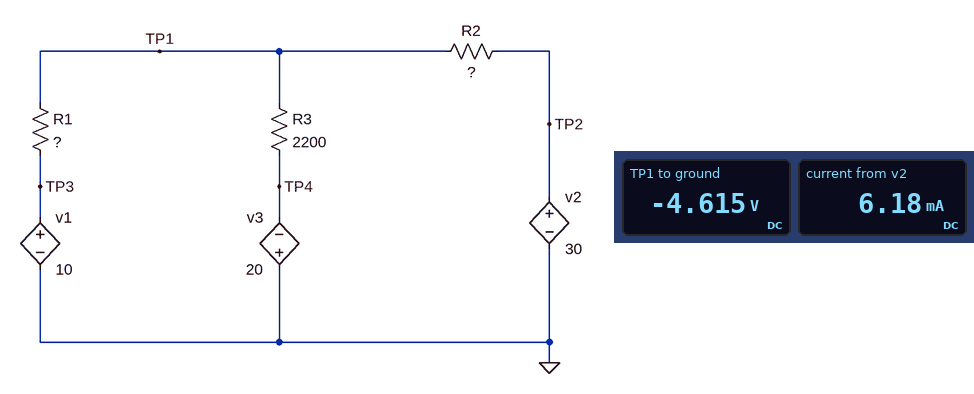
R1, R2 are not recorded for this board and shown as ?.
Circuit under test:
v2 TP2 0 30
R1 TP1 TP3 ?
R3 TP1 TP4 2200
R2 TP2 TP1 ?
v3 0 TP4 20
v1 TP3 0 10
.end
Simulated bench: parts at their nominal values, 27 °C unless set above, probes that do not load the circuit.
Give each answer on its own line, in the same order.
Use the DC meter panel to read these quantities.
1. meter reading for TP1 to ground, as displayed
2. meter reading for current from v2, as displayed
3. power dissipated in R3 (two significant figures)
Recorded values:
-4.615 V
6.18 mA
110 mW
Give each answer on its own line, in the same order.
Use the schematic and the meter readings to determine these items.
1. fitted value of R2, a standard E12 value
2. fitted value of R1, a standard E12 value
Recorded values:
5.6 kΩ
18 kΩ
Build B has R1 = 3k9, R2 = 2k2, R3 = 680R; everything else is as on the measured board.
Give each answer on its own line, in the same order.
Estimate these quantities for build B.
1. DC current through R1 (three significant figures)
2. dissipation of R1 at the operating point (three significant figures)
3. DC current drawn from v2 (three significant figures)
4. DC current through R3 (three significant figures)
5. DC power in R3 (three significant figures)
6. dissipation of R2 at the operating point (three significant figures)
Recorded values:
4.12 mA
66.1 mW
16.4 mA
20.5 mA
286 mW
591 mW
